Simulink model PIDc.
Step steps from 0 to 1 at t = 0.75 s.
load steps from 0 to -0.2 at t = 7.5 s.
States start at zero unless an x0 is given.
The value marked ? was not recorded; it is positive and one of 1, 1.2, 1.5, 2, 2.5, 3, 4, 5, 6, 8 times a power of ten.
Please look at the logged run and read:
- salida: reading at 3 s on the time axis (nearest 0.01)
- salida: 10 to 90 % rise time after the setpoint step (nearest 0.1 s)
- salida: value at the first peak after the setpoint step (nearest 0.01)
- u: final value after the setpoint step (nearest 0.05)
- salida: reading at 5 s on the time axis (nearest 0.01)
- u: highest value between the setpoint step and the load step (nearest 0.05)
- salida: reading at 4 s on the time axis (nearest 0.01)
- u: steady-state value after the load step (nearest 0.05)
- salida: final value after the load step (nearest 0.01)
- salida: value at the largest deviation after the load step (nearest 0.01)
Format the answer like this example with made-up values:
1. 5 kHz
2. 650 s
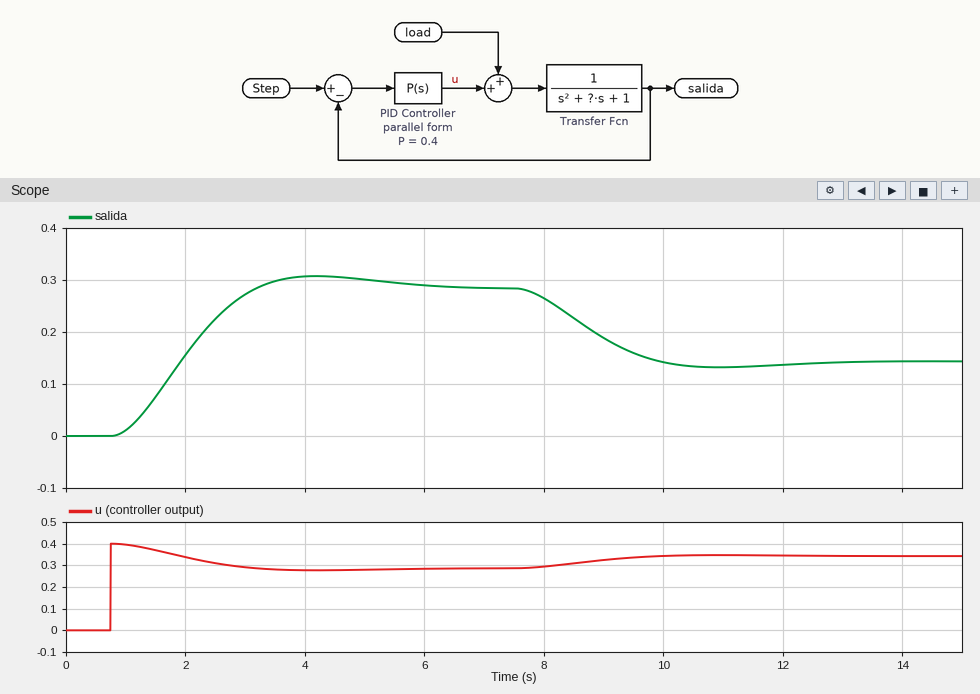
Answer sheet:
1. 0.27
2. 1.6 s
3. 0.31
4. 0.30
5. 0.30
6. 0.40
7. 0.31
8. 0.35
9. 0.14
10. 0.13
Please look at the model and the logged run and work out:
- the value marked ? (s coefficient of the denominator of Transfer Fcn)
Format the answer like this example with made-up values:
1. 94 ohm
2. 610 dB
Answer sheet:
1. 1.5
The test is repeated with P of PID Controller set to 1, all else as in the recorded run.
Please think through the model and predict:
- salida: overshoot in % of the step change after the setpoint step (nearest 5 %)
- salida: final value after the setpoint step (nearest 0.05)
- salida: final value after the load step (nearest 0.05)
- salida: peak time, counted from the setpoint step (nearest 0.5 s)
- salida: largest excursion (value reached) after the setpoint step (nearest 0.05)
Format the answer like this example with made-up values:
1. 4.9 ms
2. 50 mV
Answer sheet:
1. 15 %
2. 0.50
3. 0.40
4. 2.5 s
5. 0.55
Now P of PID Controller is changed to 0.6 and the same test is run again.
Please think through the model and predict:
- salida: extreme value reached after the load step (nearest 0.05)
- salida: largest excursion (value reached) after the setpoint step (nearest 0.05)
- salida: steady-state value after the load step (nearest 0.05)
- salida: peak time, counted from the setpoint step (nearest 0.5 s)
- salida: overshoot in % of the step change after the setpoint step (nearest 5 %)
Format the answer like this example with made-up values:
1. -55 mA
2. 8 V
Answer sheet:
1. 0.25
2. 0.40
3. 0.25
4. 3.0 s
5. 10 %
